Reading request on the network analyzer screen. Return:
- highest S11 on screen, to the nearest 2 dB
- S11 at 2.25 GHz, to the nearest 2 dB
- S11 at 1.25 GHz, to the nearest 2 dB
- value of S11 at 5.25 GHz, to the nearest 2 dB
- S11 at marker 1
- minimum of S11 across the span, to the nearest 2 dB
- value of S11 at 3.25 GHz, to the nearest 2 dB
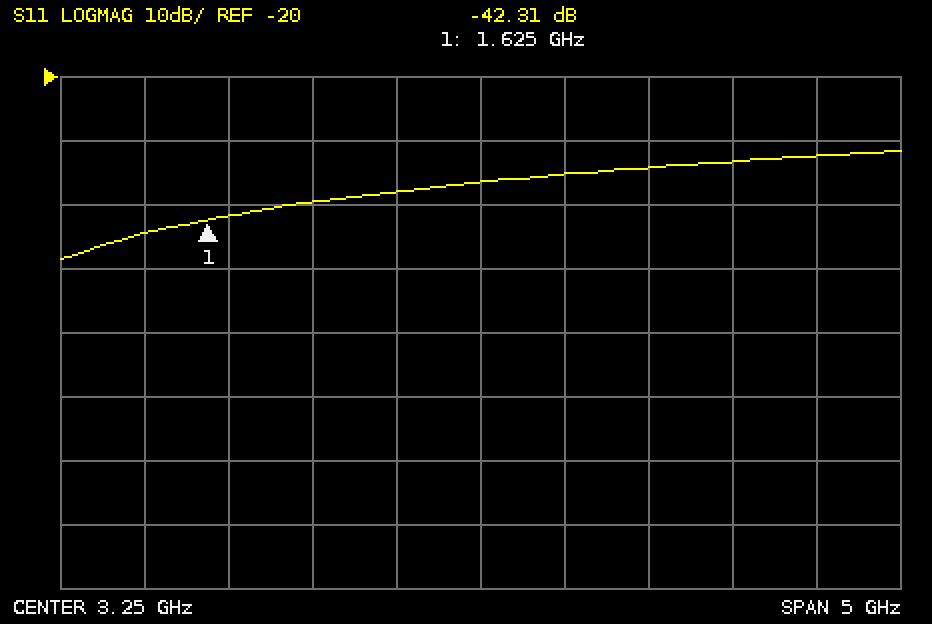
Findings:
-32 dB
-40 dB
-44 dB
-32 dB
-42.31 dB
-48 dB
-36 dB
